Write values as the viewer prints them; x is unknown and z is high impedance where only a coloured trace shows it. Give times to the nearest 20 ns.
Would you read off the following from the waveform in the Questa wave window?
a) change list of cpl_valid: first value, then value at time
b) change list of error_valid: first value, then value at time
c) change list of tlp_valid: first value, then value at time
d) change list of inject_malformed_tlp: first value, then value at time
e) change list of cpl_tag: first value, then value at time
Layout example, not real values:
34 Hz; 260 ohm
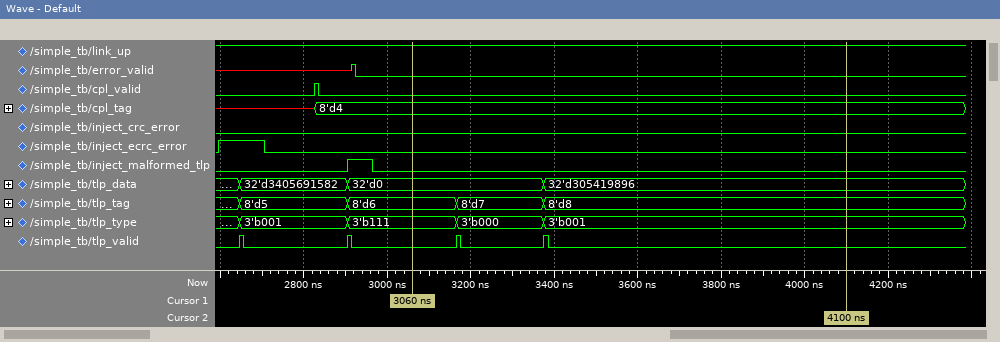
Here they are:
0, 1 at 2820 ns, 0 at 2840 ns; x, 1 at 2920 ns, 0 at 2920 ns; 0, 1 at 2640 ns, 0 at 2660 ns, 1 at 2900 ns, 0 at 2920 ns, 1 at 3160 ns, 0 at 3180 ns, 1 at 3380 ns, 0 at 3380 ns; 0, 1 at 2900 ns, 0 at 2960 ns; x, 8'd4 at 2820 ns
